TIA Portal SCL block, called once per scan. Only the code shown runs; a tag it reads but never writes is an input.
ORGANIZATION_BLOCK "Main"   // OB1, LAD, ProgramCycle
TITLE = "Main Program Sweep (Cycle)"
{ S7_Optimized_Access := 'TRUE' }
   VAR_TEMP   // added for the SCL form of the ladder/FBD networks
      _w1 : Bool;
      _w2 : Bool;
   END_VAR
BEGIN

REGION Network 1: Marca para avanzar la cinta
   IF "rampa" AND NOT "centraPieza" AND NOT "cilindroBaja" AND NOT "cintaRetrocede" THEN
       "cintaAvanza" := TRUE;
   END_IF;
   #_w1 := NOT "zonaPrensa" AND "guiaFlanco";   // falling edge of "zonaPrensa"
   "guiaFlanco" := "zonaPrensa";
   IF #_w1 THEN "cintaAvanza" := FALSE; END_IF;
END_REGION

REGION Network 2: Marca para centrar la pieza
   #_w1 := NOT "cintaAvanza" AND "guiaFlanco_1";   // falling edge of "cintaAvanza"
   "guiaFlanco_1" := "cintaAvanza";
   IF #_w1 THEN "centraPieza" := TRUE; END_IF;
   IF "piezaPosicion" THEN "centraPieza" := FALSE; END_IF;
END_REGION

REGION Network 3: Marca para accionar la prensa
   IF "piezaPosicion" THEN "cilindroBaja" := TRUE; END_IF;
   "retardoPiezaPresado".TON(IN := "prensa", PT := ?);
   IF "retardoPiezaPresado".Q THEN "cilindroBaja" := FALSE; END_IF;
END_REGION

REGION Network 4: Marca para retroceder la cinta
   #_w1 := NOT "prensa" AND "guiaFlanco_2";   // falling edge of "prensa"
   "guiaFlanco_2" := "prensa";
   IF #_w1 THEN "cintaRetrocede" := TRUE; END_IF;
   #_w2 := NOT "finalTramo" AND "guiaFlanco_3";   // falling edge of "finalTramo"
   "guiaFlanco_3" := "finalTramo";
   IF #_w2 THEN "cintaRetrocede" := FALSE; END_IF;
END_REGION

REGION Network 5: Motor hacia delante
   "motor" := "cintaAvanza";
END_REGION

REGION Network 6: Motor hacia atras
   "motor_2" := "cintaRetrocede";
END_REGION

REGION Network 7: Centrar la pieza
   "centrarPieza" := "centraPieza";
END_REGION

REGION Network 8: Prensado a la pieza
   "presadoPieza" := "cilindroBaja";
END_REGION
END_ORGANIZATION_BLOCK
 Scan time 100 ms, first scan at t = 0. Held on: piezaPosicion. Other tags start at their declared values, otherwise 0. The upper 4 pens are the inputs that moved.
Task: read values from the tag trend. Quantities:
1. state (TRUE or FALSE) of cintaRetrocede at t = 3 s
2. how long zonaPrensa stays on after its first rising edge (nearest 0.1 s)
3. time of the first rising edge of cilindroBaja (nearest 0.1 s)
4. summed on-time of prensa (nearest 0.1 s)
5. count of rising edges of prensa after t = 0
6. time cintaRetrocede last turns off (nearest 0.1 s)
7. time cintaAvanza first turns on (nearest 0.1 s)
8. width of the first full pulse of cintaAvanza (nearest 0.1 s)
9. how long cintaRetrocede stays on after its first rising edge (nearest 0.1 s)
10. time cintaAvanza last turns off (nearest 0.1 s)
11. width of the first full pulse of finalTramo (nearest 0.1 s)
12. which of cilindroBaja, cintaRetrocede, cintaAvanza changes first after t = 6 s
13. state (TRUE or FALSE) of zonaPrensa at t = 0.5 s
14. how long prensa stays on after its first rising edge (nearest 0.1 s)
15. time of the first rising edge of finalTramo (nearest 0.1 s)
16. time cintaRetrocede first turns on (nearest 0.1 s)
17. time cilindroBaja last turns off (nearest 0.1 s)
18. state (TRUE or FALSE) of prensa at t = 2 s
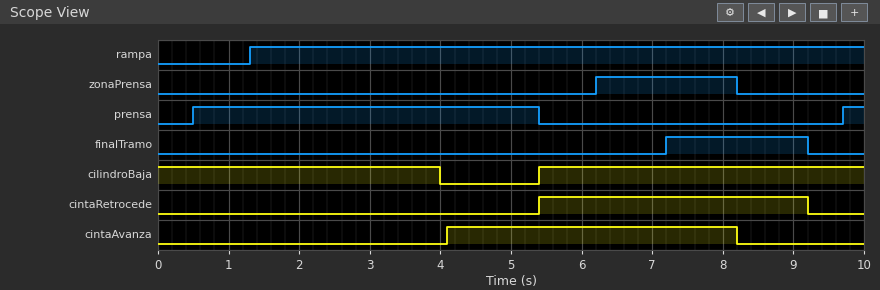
FALSE
2.0 s
5.4 s
5.2 s
2
9.2 s
4.1 s
4.1 s
3.8 s
8.2 s
2.0 s
cintaAvanza
FALSE
4.9 s
7.2 s
5.4 s
4.0 s
TRUE
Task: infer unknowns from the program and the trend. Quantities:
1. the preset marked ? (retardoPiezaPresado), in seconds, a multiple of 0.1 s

3.5 s
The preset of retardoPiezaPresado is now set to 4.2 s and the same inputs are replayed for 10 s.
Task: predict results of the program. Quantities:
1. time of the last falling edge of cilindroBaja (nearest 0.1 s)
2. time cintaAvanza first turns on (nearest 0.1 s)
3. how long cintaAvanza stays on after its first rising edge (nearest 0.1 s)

4.7 s
4.8 s
3.4 s
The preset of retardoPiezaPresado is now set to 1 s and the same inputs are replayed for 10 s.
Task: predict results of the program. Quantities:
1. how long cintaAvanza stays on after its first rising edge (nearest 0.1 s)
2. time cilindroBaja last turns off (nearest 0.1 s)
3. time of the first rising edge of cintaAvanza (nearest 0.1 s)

6.6 s
1.5 s
1.6 s
